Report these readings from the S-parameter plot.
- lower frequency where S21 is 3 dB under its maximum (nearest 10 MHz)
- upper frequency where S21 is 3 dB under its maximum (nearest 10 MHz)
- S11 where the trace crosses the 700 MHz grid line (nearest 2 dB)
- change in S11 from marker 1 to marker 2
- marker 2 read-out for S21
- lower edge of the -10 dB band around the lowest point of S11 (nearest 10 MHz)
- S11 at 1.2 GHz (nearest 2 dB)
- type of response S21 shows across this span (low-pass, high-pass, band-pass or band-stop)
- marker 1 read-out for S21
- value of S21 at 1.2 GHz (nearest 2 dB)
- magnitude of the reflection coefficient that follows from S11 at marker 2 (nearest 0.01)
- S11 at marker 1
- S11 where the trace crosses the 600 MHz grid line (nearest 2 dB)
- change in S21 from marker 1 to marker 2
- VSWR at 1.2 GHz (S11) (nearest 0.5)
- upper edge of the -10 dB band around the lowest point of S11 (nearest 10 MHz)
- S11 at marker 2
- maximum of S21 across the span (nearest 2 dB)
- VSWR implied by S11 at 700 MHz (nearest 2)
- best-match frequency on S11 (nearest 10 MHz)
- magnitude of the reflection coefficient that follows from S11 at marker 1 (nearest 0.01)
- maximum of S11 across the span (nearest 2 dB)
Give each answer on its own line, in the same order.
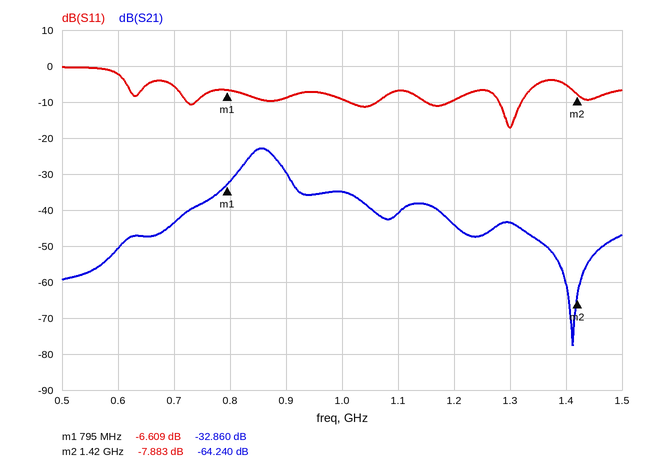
830 MHz
880 MHz
-6 dB
-1.274 dB
-64.240 dB
1.28 GHz
-10 dB
band-pass
-32.860 dB
-44 dB
0.40
-6.609 dB
-2 dB
-31.380 dB
2.0
1.32 GHz
-7.883 dB
-22 dB
4
1.30 GHz
0.47
0 dB
